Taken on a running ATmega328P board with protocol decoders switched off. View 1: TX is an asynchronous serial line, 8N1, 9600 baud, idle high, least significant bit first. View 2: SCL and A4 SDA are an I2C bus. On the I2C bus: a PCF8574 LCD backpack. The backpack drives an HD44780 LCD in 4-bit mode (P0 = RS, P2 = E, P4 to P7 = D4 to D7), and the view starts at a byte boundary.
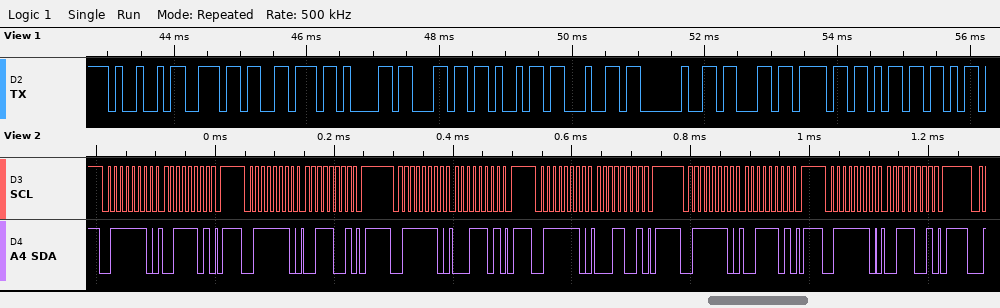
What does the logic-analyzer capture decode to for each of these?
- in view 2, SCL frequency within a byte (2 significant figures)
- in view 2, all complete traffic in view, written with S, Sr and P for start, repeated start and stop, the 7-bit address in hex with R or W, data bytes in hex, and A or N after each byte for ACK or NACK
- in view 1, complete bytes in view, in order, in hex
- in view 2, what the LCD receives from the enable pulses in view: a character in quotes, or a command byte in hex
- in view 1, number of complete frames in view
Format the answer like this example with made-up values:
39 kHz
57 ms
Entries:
100 kHz
S 3FW A 3D A P S 3FW A 39 A P S 3FW A 1D A P S 3FW A 19 A P S 3FW A 3D A P S 3FW A 39 A P
49 6E 76 61 6C 69 64 20 63 6F 6D
'1'
11
